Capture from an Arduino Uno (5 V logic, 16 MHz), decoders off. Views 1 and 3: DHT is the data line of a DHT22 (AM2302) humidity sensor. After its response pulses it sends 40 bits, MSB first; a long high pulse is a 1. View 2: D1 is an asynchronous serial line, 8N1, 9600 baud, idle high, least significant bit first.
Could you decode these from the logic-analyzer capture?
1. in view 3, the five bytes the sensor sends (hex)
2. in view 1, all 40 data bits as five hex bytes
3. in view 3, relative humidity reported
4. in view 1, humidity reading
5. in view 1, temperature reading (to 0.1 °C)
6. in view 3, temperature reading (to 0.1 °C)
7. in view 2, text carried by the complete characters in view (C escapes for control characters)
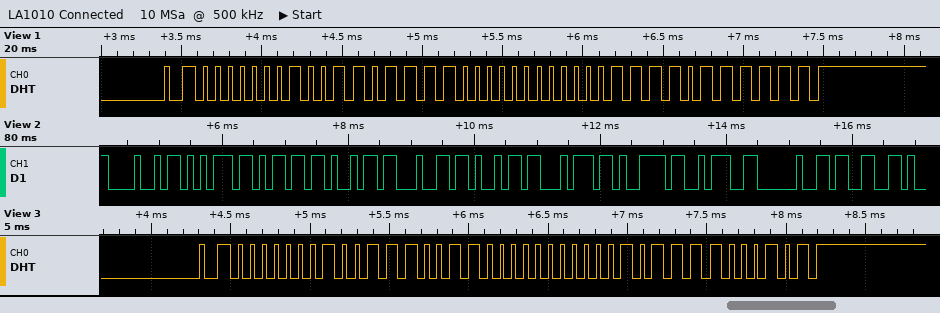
01 39 80 0B C5
01 37 80 07 BF
31.3 %
31.1 %
-0.7 °C
-1.1 °C
"Humidity: 3"
